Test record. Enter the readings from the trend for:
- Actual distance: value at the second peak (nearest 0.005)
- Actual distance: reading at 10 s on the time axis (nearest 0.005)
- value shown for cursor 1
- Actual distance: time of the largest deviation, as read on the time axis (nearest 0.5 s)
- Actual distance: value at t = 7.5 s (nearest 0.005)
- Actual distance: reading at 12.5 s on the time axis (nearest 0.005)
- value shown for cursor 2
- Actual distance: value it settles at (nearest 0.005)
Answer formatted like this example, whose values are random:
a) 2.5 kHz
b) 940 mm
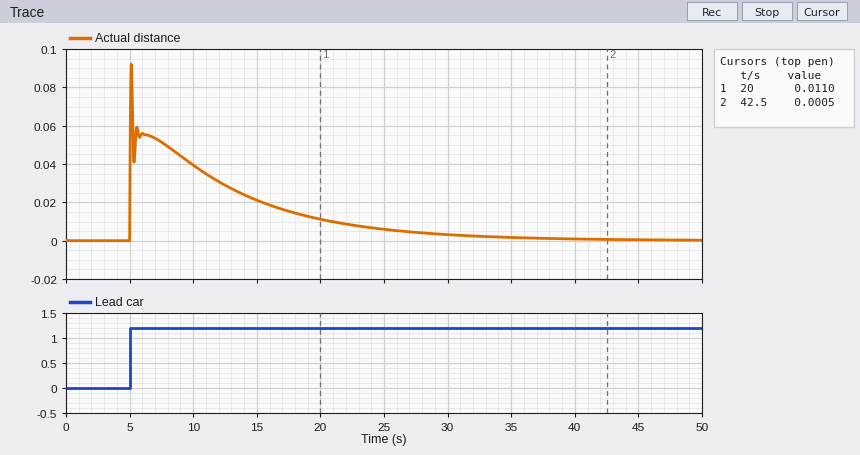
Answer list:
a) 0.060
b) 0.040
c) 0.0110
d) 5.0 s
e) 0.050
f) 0.030
g) 0.0005
h) 0.000
